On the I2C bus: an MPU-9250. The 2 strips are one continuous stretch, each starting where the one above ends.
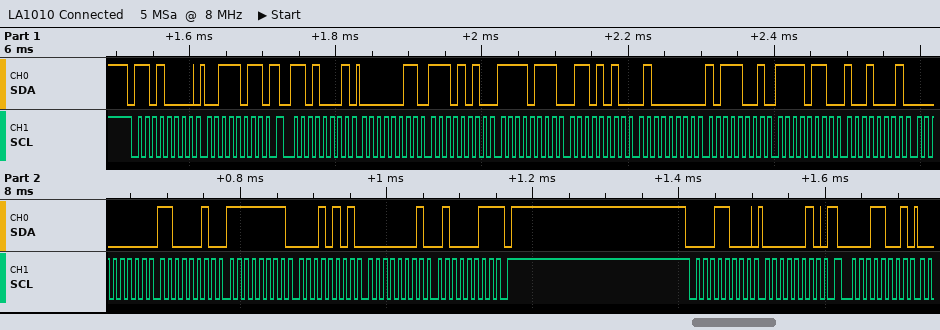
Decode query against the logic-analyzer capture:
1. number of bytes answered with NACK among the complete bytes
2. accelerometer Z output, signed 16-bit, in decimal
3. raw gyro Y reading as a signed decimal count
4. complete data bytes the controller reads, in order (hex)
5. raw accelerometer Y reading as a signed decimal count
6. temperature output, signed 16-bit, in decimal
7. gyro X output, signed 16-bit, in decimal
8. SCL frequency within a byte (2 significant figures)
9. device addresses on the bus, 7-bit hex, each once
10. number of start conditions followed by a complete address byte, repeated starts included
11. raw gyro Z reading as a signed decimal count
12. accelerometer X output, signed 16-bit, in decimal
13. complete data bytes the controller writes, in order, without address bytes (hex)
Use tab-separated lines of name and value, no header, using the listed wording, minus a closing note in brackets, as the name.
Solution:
number of bytes answered with NACK among the complete bytes	1
accelerometer Z output, signed 16-bit, in decimal	16569
raw gyro Y reading as a signed decimal count	-235
complete data bytes the controller reads, in order	03 EA F7 6A 40 B9 F6 91 00 C2 FF 15 01 43
raw accelerometer Y reading as a signed decimal count	-2198
temperature output, signed 16-bit, in decimal	-2415
gyro X output, signed 16-bit, in decimal	194
SCL frequency within a byte	100 kHz
device addresses on the bus, 7-bit hex, each once	0x68 0x0C
number of start conditions followed by a complete address byte, repeated starts included	4
raw gyro Z reading as a signed decimal count	323
accelerometer X output, signed 16-bit, in decimal	1002
complete data bytes the controller writes, in order, without address bytes	3B 02
